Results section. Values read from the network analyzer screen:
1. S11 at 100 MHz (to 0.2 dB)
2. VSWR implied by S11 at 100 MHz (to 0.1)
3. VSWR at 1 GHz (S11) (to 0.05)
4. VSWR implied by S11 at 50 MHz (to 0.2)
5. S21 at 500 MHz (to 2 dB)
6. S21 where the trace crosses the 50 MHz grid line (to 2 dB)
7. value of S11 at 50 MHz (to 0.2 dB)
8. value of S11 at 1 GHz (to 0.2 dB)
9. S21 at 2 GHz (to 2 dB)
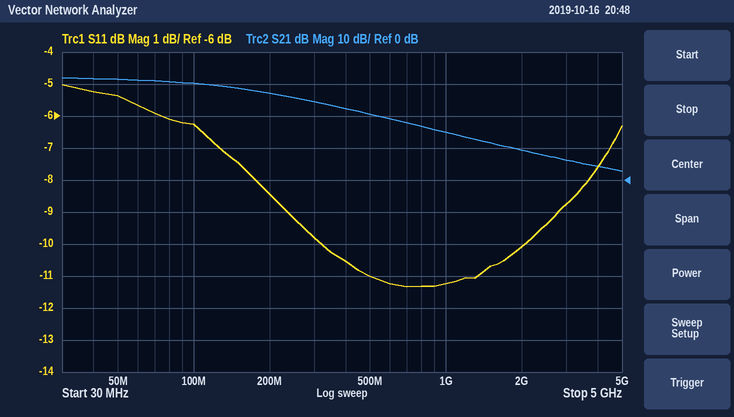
-6.2 dB
2.9
1.75
3.4
20 dB
32 dB
-5.4 dB
-11.2 dB
10 dB
